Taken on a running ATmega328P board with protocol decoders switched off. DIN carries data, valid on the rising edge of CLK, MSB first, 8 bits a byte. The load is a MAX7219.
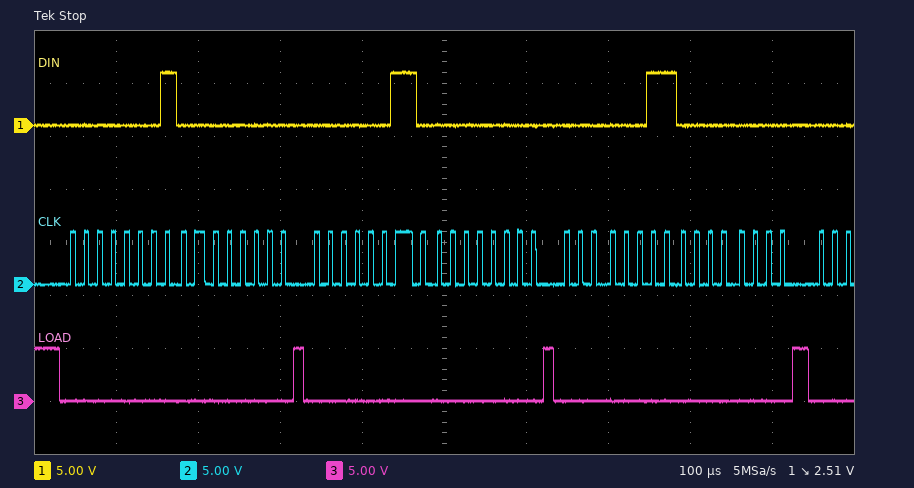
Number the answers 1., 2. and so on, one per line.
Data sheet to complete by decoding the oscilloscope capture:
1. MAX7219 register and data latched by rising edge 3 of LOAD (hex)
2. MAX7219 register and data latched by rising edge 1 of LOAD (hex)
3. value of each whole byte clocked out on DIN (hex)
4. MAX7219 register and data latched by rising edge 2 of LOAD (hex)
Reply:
1. register 0x3, data 0x00
2. register 0x1, data 0x00
3. 01 00 02 00 03 00
4. register 0x2, data 0x00
